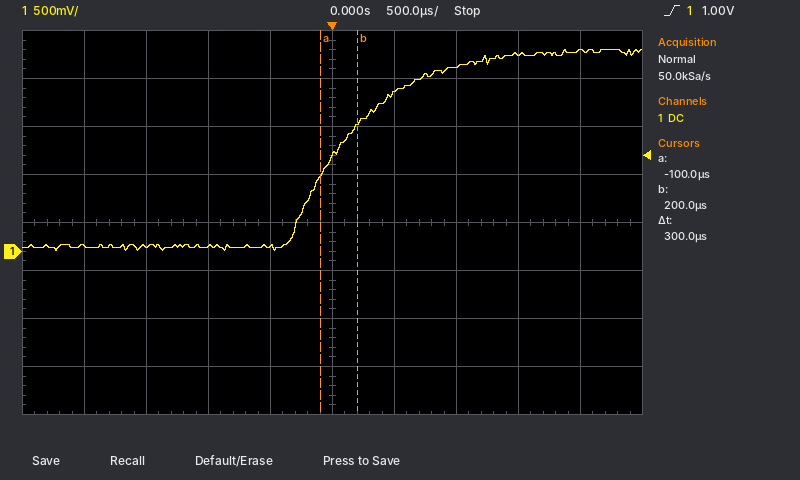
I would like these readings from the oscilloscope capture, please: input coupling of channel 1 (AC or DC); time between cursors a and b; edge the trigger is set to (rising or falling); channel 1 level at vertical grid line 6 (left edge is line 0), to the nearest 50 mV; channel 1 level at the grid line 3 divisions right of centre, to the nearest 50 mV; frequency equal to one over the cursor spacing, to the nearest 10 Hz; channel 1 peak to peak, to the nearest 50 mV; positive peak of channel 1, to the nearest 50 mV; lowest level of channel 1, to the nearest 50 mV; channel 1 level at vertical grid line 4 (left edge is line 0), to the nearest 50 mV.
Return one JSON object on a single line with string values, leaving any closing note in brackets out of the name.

{"input coupling of channel 1": "DC", "time between cursors a and b": "300 µs", "edge the trigger is set to": "rising", "channel 1 level at vertical grid line 6 (left edge is line 0), to the nearest 50 mV": "1.65 V", "channel 1 level at the grid line 3 divisions right of centre, to the nearest 50 mV": "2.05 V", "frequency equal to one over the cursor spacing, to the nearest 10 Hz": "3.33 kHz", "channel 1 peak to peak, to the nearest 50 mV": "2.10 V", "positive peak of channel 1, to the nearest 50 mV": "2.10 V", "lowest level of channel 1, to the nearest 50 mV": "0 mV", "channel 1 level at vertical grid line 4 (left edge is line 0), to the nearest 50 mV": "50 mV"}
